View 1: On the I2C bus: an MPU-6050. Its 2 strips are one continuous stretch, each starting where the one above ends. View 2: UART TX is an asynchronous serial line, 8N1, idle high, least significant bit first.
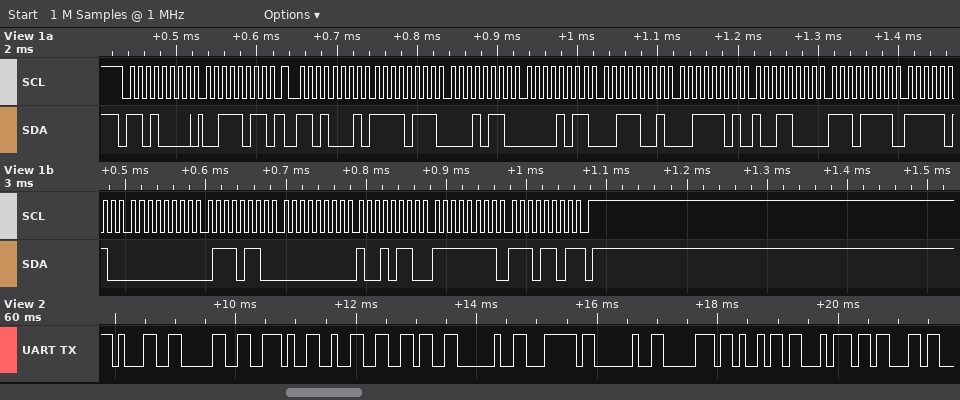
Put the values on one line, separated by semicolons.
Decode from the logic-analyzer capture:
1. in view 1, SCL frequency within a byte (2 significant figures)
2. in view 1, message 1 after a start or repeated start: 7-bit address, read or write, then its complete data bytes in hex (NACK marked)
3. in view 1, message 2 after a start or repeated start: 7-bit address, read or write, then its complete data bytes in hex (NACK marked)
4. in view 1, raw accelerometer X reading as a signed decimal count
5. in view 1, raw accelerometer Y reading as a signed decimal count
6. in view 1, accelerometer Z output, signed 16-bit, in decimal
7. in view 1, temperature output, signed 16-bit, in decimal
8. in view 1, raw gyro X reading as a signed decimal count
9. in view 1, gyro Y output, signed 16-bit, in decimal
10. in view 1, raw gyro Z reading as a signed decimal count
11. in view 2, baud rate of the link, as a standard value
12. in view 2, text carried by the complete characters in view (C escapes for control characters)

100 kHz; 0x68 write: 3B; 0x68 read: F7 16 0B 39 3D 98 EF FA 00 76 00 96 FF ED NACK; -2282; 2873; 15768; -4102; 118; 150; -19; 9600 baud; "10.26 | pitc"
